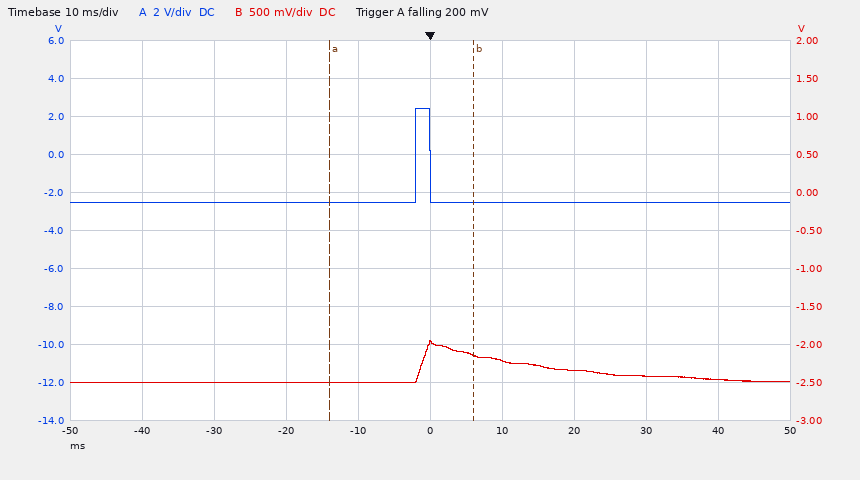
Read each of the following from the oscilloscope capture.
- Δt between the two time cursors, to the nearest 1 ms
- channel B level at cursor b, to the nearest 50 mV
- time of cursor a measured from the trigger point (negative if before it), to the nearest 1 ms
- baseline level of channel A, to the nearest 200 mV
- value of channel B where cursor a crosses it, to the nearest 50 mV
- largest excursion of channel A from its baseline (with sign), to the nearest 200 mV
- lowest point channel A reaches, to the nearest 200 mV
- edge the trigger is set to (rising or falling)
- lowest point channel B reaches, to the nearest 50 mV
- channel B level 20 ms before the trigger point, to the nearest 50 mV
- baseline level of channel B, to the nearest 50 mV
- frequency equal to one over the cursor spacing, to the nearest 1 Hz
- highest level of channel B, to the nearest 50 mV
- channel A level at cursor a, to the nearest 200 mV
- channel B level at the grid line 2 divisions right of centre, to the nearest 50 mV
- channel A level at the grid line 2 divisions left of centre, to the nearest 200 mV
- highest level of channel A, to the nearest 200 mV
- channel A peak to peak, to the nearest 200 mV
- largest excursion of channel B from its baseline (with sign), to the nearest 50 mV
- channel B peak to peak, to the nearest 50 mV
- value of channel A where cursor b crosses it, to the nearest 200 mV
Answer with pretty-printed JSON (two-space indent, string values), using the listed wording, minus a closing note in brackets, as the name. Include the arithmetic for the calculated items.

{
  "Δt between the two time cursors, to the nearest 1 ms": "20 ms",
  "channel B level at cursor b, to the nearest 50 mV": "-2.15 V",
  "time of cursor a measured from the trigger point (negative if before it), to the nearest 1 ms": "-14 ms",
  "baseline level of channel A, to the nearest 200 mV": "-2.6 V",
  "value of channel B where cursor a crosses it, to the nearest 50 mV": "-2.50 V",
  "largest excursion of channel A from its baseline (with sign), to the nearest 200 mV": "2.4 V − (-2.6 V) = +5.0 V",
  "lowest point channel A reaches, to the nearest 200 mV": "-2.6 V",
  "edge the trigger is set to": "falling",
  "lowest point channel B reaches, to the nearest 50 mV": "-2.50 V",
  "channel B level 20 ms before the trigger point, to the nearest 50 mV": "-2.50 V",
  "baseline level of channel B, to the nearest 50 mV": "-2.50 V",
  "frequency equal to one over the cursor spacing, to the nearest 1 Hz": "1 / 20 ms ≈ 50 Hz",
  "highest level of channel B, to the nearest 50 mV": "-1.95 V",
  "channel A level at cursor a, to the nearest 200 mV": "-2.6 V",
  "channel B level at the grid line 2 divisions right of centre, to the nearest 50 mV": "-2.35 V",
  "channel A level at the grid line 2 divisions left of centre, to the nearest 200 mV": "-2.6 V",
  "highest level of channel A, to the nearest 200 mV": "2.4 V",
  "channel A peak to peak, to the nearest 200 mV": "2.4 V − (-2.6 V) = 5.0 V",
  "largest excursion of channel B from its baseline (with sign), to the nearest 50 mV": "-1.95 V − (-2.50 V) = +550 mV",
  "channel B peak to peak, to the nearest 50 mV": "-1.95 V − (-2.50 V) = 550 mV",
  "value of channel A where cursor b crosses it, to the nearest 200 mV": "-2.6 V"
}
